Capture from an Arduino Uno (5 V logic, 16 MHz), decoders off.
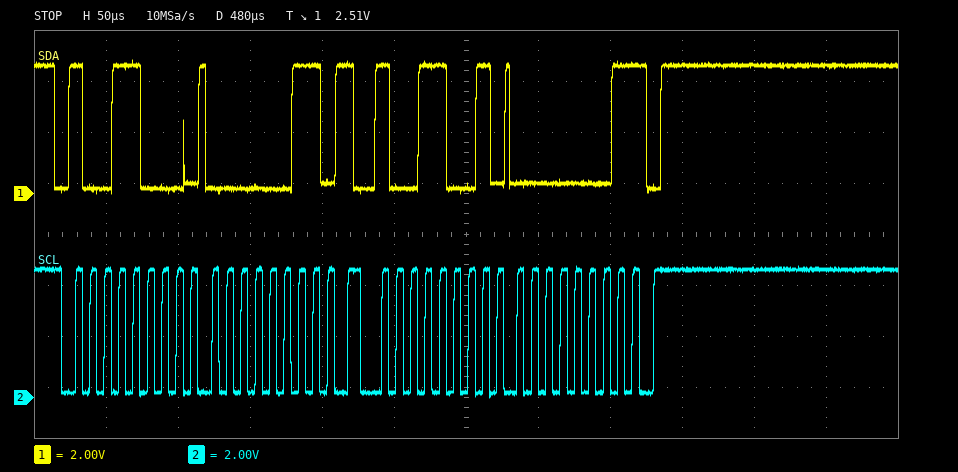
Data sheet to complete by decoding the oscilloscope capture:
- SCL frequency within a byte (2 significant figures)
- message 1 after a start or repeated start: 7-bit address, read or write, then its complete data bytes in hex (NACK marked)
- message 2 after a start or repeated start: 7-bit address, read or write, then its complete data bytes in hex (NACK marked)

100 kHz
0x4C write: 03
0x4C read: 01 NACK
